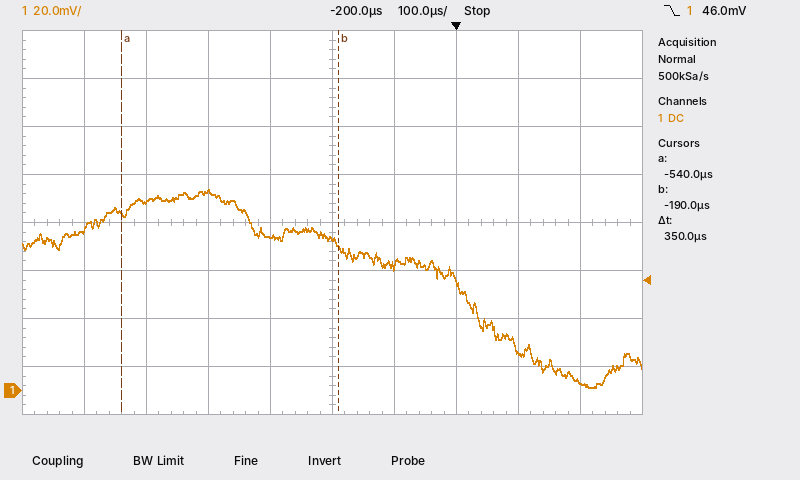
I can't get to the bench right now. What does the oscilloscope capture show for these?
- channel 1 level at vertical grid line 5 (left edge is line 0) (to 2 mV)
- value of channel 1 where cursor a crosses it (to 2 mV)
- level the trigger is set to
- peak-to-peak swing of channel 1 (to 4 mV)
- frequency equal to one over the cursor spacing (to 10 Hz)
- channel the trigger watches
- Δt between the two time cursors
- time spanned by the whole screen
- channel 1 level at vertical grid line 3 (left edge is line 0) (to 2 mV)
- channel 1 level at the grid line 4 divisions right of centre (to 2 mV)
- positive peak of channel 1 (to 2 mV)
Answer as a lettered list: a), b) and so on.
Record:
a) 64 mV
b) 74 mV
c) 46.0 mV
d) 84 mV
e) 2.86 kHz
f) channel 1
g) 350 µs
h) 1 ms
i) 82 mV
j) 4 mV
k) 84 mV
